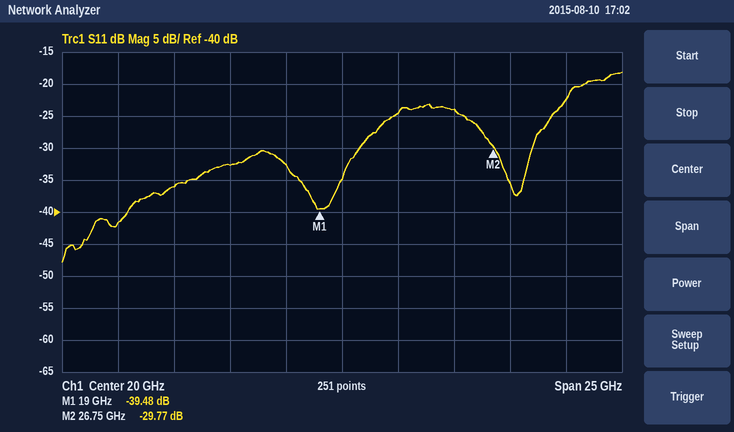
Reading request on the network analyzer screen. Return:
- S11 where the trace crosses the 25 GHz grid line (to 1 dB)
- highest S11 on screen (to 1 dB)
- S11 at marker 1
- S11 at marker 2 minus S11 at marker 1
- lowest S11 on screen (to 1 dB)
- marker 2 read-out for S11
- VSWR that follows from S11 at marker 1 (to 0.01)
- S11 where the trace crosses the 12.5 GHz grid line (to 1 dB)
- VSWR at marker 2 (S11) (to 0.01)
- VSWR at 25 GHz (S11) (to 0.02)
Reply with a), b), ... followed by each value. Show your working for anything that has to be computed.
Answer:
a) -24 dB
b) -18 dB
c) -39.48 dB
d) -29.77 − (-39.48) = 9.71 dB
e) -48 dB
f) -29.77 dB
g) (1 + 0.0106)/(1 − 0.0106) ≈ 1.02
h) -36 dB
i) (1 + 0.0325)/(1 − 0.0325) ≈ 1.07
j) |Γ| = 10^(-24/20) = 0.0631; VSWR = (1 + 0.0631)/(1 − 0.0631) ≈ 1.13, so 1.14 to the nearest 0.02
